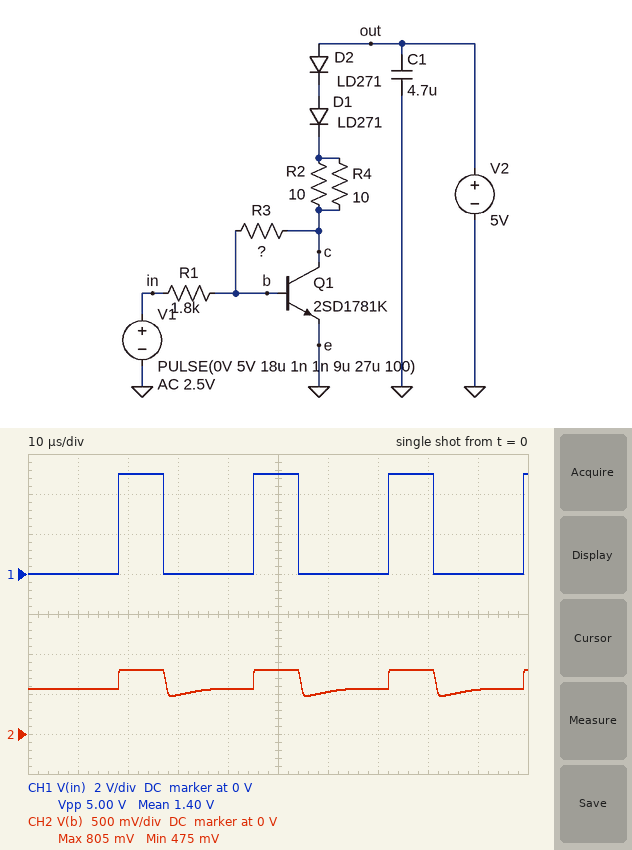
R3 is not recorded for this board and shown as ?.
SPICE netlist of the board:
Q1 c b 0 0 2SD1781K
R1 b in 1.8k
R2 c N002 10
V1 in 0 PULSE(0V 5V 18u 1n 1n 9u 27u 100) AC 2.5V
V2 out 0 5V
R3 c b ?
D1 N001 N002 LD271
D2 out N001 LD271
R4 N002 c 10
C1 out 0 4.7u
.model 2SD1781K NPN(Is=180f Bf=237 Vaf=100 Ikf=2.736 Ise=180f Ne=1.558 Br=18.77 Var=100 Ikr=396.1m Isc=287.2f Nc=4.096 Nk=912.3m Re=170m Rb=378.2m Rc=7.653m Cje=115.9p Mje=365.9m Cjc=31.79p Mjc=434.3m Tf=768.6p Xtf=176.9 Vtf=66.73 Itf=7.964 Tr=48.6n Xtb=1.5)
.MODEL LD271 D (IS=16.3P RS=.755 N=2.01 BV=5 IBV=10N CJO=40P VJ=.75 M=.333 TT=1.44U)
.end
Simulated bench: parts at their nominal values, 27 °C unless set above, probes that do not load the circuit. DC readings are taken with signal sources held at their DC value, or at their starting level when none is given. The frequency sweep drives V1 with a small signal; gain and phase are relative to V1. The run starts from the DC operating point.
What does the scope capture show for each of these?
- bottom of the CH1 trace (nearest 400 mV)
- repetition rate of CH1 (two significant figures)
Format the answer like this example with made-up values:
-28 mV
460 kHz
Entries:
0 V
37 kHz
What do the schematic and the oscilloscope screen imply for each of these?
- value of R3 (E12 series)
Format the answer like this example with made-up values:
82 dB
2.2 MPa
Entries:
8.2 kΩ
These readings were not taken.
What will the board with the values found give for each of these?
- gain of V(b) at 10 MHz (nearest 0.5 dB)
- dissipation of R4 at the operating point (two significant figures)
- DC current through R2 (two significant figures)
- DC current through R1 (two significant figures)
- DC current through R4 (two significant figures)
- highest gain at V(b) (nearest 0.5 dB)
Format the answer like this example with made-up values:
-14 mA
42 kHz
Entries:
-27.5 dB
1.8 µW
420 µA
310 µA
420 µA
-4.0 dB
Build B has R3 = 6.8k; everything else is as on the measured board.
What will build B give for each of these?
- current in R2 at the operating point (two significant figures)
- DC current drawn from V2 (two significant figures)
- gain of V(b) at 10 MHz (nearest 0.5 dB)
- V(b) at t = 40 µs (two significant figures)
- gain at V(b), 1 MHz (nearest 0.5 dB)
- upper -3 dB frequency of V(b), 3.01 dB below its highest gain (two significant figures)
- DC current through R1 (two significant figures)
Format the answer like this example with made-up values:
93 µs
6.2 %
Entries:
1.6 mA
3.3 mA
-30.5 dB
610 mV
-12.0 dB
860 kHz
340 µA
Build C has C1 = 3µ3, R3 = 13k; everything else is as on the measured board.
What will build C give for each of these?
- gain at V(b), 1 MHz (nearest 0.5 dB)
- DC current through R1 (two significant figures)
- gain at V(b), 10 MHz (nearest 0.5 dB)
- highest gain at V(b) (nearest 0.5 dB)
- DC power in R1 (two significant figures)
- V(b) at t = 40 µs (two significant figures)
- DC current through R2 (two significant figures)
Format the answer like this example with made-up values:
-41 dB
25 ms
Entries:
-7.0 dB
220 µA
-25.5 dB
-1.0 dB
89 µW
400 mV
110 µA
